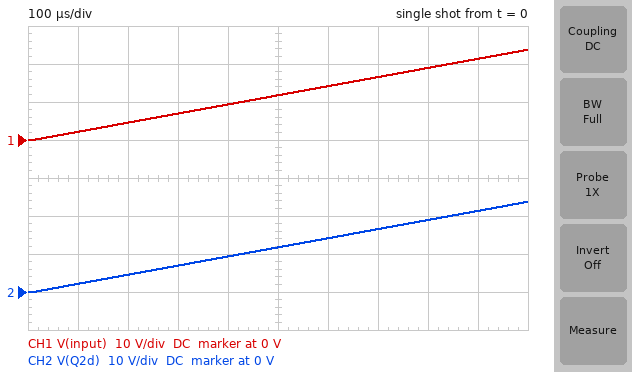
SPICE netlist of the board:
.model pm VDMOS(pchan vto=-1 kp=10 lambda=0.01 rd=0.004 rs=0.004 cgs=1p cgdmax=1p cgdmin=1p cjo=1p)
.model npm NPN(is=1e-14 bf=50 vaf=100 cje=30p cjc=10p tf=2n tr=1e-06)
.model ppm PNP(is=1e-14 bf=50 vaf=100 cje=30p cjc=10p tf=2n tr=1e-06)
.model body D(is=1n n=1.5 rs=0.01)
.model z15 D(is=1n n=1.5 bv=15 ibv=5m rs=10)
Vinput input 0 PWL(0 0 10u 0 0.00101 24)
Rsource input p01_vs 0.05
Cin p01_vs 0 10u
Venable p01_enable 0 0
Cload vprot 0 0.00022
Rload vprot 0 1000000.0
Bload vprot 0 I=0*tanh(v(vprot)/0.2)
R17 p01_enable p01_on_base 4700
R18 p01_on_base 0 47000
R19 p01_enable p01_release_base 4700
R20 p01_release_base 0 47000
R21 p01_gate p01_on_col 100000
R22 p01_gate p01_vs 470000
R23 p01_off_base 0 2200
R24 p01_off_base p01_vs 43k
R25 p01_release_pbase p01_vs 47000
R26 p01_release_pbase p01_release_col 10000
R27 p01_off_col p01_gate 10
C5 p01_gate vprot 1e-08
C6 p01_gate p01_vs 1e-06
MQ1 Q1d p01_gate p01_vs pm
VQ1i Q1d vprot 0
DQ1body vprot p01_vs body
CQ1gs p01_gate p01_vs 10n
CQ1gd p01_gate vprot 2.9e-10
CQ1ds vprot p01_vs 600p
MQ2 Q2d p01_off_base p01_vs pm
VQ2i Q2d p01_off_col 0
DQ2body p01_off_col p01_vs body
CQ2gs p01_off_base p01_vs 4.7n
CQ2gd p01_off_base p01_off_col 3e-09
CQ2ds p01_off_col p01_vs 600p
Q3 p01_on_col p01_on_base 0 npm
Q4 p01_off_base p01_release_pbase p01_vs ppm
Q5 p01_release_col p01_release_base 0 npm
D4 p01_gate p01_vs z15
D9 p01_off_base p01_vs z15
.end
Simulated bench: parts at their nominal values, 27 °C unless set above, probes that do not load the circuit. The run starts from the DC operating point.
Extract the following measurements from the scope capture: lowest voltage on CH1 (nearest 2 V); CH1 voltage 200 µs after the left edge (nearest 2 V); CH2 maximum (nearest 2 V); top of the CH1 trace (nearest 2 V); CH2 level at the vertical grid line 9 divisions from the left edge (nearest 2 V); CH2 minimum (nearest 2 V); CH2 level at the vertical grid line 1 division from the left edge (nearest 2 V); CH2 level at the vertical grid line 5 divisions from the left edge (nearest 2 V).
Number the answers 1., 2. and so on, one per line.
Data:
1. 0 V
2. 4 V
3. 24 V
4. 24 V
5. 22 V
6. 0 V
7. 2 V
8. 12 V
